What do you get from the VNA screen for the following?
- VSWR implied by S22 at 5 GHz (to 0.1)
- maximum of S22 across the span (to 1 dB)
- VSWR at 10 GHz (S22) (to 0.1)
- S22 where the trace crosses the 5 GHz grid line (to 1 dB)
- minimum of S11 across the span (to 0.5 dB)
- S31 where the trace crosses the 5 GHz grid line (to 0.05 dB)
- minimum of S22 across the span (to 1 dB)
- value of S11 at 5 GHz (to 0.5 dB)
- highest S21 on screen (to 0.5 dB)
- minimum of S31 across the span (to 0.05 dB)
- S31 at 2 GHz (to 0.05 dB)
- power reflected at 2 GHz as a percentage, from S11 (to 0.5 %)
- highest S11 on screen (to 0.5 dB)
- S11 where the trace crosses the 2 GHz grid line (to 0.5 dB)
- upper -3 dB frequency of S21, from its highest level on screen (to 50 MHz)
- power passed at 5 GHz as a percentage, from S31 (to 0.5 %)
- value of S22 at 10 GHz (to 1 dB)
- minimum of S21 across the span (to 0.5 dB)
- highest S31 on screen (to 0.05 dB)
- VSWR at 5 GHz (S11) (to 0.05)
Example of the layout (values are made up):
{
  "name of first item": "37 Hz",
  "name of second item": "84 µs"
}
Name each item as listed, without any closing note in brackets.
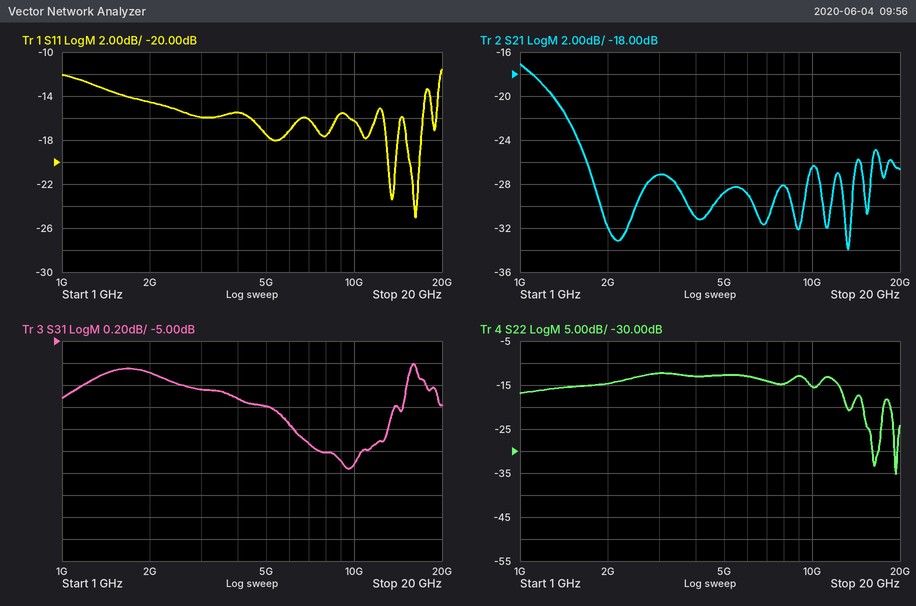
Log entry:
{
  "VSWR implied by S22 at 5 GHz": "1.6",
  "maximum of S22 across the span": "-12 dB",
  "VSWR at 10 GHz (S22)": "1.4",
  "S22 where the trace crosses the 5 GHz grid line": "-13 dB",
  "minimum of S11 across the span": "-25.0 dB",
  "S31 where the trace crosses the 5 GHz grid line": "-5.60 dB",
  "minimum of S22 across the span": "-35 dB",
  "value of S11 at 5 GHz": "-17.5 dB",
  "highest S21 on screen": "-17.0 dB",
  "minimum of S31 across the span": "-6.15 dB",
  "S31 at 2 GHz": "-5.30 dB",
  "power reflected at 2 GHz as a percentage, from S11": "3.5 %",
  "highest S11 on screen": "-11.5 dB",
  "S11 where the trace crosses the 2 GHz grid line": "-14.5 dB",
  "upper -3 dB frequency of S21, from its highest level on screen": "1.30 GHz",
  "power passed at 5 GHz as a percentage, from S31": "27.5 %",
  "value of S22 at 10 GHz": "-15 dB",
  "minimum of S21 across the span": "-34.0 dB",
  "highest S31 on screen": "-5.20 dB",
  "VSWR at 5 GHz (S11)": "1.30"
}
